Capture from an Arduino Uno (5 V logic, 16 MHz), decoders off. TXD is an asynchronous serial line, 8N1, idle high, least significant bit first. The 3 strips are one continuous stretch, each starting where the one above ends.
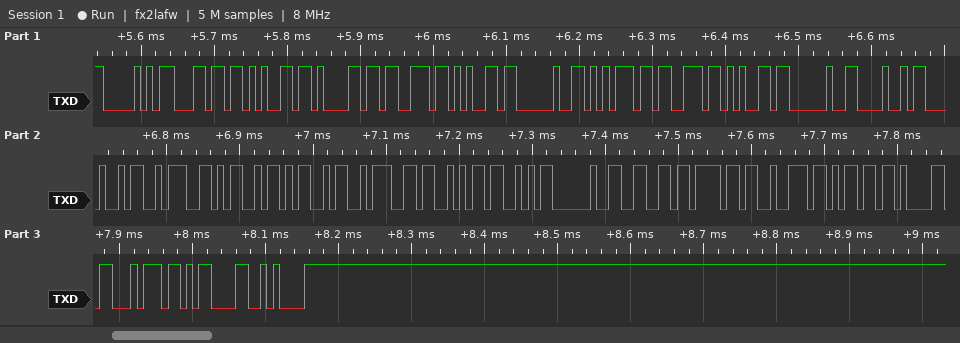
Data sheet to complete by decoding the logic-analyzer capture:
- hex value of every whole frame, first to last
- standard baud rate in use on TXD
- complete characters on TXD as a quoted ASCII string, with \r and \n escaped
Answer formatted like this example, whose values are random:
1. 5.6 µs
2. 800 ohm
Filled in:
1. 50 6C 65 61 73 65 20 75 73 65 20 48 48 3A 4D 4D 3A 53 53 20 66 6F 72 6D 61 74 0D 0A
2. 115200 baud
3. "Please use HH:MM:SS format\r\n"
